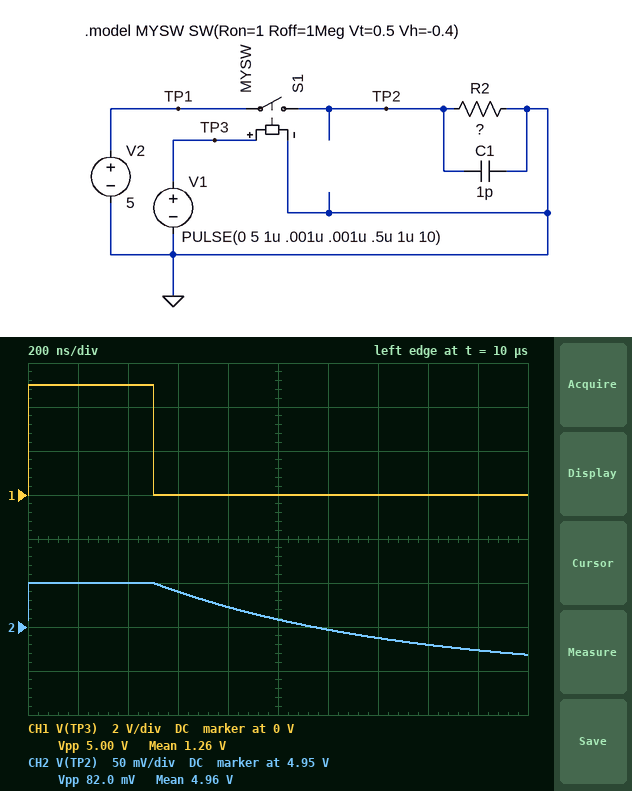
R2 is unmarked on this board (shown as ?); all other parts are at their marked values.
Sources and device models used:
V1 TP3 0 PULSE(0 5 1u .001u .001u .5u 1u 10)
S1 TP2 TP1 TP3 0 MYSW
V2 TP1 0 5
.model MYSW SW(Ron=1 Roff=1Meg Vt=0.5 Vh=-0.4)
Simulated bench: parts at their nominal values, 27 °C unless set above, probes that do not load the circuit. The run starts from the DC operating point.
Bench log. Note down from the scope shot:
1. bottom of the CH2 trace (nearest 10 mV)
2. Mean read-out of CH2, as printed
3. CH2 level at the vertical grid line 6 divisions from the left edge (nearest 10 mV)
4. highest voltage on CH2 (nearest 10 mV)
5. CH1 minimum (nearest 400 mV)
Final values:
4.92 V
4.96 V
4.95 V
5.00 V
0 V
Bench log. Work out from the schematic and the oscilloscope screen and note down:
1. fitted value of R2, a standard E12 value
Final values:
47 MΩ
